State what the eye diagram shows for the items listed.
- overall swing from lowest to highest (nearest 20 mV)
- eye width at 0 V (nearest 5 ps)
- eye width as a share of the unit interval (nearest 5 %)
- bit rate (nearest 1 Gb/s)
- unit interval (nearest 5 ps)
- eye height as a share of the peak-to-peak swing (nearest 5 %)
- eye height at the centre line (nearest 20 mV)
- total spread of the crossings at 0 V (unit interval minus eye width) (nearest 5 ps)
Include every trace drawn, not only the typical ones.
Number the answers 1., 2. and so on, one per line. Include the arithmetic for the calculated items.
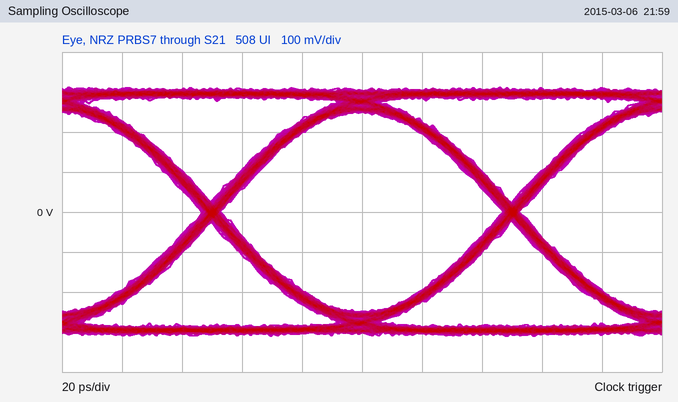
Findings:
1. 620 mV
2. 95 ps
3. 95 ps / 100 ps ≈ 95 %
4. 10 Gb/s
5. 100 ps
6. 500 mV / 620 mV ≈ 80.6 %, so 80 % to the nearest 5 %
7. 500 mV
8. 5 ps
